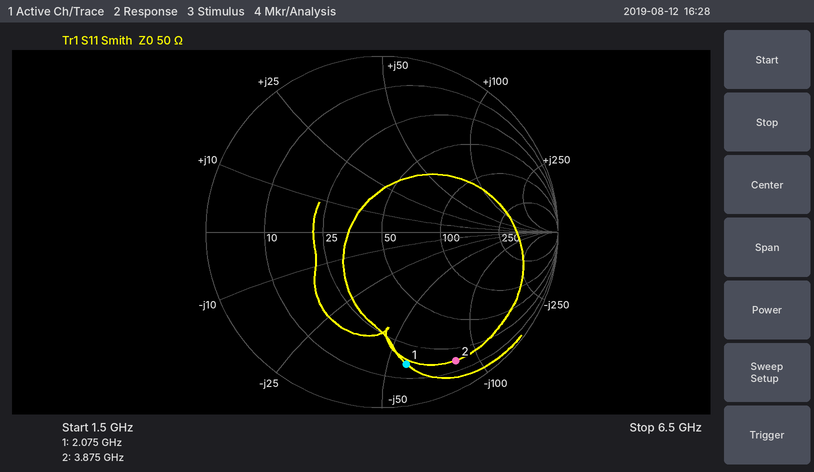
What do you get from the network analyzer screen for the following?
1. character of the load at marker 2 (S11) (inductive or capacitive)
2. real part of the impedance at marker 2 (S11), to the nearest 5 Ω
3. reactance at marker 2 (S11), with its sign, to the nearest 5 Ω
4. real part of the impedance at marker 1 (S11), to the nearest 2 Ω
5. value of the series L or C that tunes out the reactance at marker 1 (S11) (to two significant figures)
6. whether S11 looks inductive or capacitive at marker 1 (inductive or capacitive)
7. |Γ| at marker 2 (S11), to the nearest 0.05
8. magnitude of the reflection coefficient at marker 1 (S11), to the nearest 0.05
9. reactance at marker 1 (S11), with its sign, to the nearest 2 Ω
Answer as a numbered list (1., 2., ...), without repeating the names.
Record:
1. capacitive
2. 15 Ω
3. -85 Ω
4. 16 Ω
5. 4.4 nH
6. capacitive
7. 0.85
8. 0.75
9. -58 Ω
